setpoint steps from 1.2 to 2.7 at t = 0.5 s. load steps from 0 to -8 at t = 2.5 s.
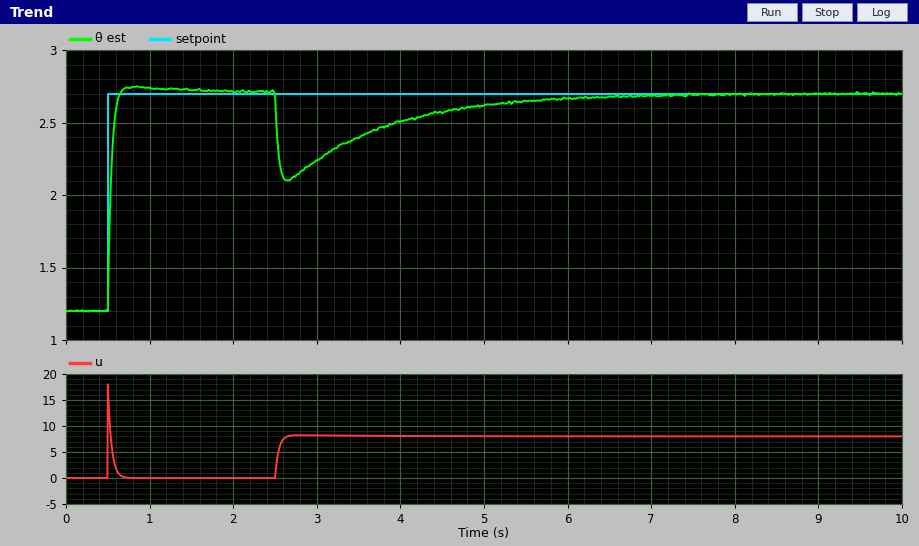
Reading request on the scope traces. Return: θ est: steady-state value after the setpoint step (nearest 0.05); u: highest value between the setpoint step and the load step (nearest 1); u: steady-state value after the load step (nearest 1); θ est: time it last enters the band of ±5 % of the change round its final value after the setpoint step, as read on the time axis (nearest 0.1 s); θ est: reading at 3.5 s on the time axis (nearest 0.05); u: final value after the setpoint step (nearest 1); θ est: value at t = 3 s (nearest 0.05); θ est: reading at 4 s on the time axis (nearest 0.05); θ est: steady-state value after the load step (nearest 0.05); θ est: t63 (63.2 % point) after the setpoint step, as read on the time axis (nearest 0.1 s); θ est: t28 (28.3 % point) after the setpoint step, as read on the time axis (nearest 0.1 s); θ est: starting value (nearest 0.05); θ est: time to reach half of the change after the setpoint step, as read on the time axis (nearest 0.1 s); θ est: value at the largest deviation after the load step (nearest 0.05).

2.70
18
8
0.6 s
2.40
0
2.25
2.50
2.70
0.5 s
0.5 s
1.20
0.5 s
2.10
